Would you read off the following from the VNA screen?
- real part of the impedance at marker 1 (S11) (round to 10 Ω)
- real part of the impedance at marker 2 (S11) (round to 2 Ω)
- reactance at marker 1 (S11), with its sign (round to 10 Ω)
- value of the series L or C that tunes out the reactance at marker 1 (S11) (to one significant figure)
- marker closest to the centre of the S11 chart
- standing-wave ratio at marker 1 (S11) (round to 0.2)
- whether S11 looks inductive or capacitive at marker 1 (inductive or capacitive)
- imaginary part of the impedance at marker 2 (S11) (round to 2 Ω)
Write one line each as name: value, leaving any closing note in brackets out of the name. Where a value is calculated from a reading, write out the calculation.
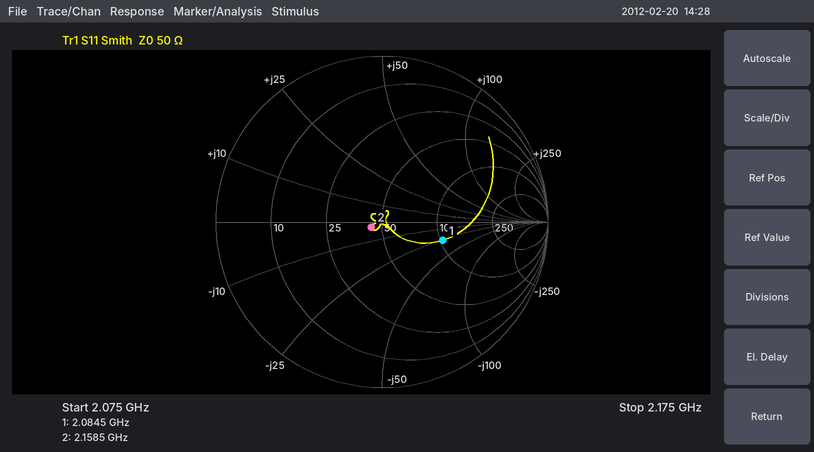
real part of the impedance at marker 1 (S11): 100 Ω
real part of the impedance at marker 2 (S11): 44 Ω
reactance at marker 1 (S11), with its sign: -30 Ω
value of the series L or C that tunes out the reactance at marker 1 (S11): L = 30 Ω/(2π × 2.0845 GHz) ≈ 2 nH
marker closest to the centre of the S11 chart: marker 2
standing-wave ratio at marker 1 (S11): 2.2
whether S11 looks inductive or capacitive at marker 1: capacitive
imaginary part of the impedance at marker 2 (S11): -2 Ω
